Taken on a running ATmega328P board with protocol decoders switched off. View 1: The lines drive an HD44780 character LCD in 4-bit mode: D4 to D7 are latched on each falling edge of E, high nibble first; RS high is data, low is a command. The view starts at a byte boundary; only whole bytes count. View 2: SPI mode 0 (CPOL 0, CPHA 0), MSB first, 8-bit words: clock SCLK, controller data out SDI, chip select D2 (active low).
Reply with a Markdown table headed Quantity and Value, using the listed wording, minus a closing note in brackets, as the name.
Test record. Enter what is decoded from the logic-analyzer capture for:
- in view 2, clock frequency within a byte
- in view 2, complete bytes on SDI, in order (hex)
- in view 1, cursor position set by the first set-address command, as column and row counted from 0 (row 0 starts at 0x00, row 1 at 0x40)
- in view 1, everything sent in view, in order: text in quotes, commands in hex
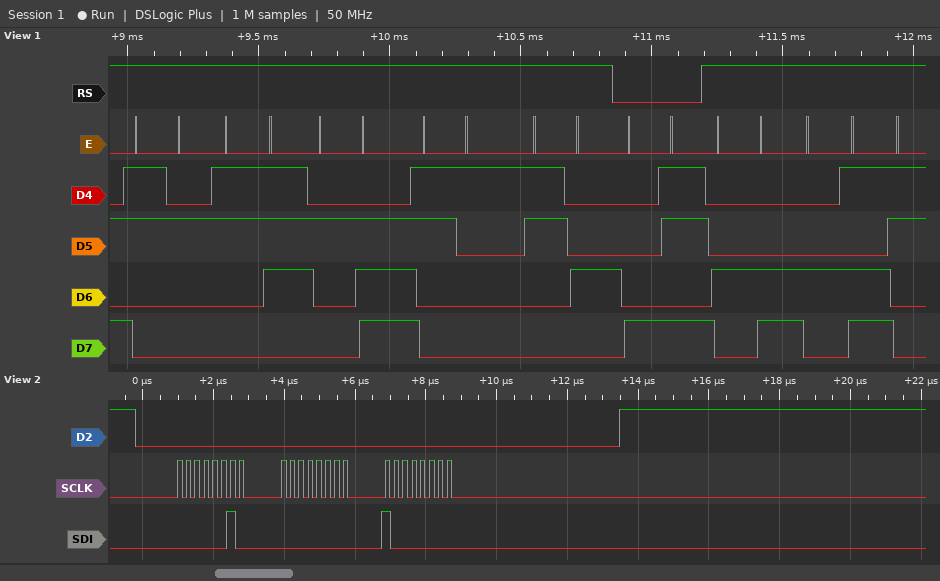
| Quantity | Value |
|---|---|
| in view 2, clock frequency within a byte | 4 MHz |
| in view 2, complete bytes on SDI, in order | 02 00 80 |
| in view 1, cursor position set by the first set-address command, as column and row counted from 0 | column 11, row 0 |
| in view 1, everything sent in view, in order: text in quotes, commands in hex | "27.14" 0x8B "LM" |
